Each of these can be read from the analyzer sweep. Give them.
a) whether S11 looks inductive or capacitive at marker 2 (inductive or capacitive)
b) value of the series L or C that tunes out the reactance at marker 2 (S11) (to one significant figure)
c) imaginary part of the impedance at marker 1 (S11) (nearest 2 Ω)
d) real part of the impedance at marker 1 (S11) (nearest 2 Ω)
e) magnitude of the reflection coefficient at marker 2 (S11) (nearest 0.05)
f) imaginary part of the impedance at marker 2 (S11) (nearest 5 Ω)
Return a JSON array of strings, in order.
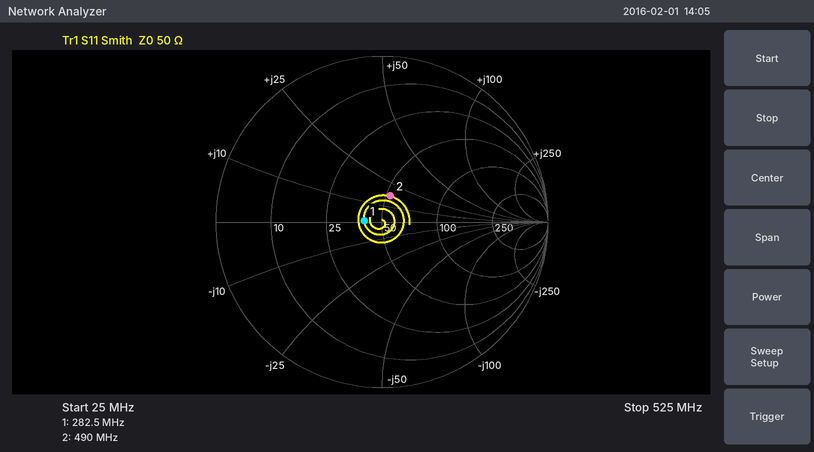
["inductive", "20 pF", "0 Ω", "40 Ω", "0.15", "+15 Ω"]
